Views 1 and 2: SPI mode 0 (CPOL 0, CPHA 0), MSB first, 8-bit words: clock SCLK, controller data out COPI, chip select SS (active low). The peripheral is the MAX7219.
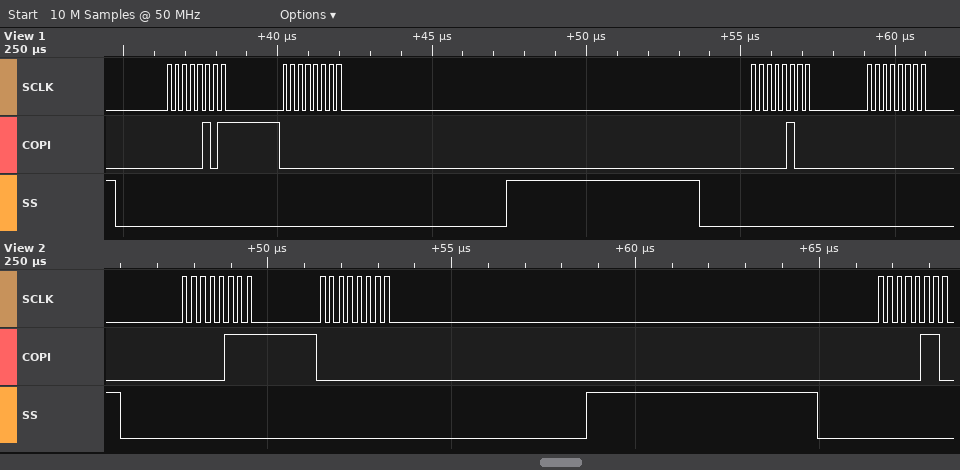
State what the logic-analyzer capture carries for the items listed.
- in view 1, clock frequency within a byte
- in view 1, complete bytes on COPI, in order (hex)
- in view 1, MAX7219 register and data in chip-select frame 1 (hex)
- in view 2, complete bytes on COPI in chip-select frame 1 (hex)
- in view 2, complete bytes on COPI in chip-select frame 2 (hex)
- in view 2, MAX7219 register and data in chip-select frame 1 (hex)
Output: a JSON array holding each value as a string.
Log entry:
["4 MHz", "0x05 0x00 0x04 0x00", "register 0x5, data 0x00", "07 00", "06", "register 0x7, data 0x00"]
